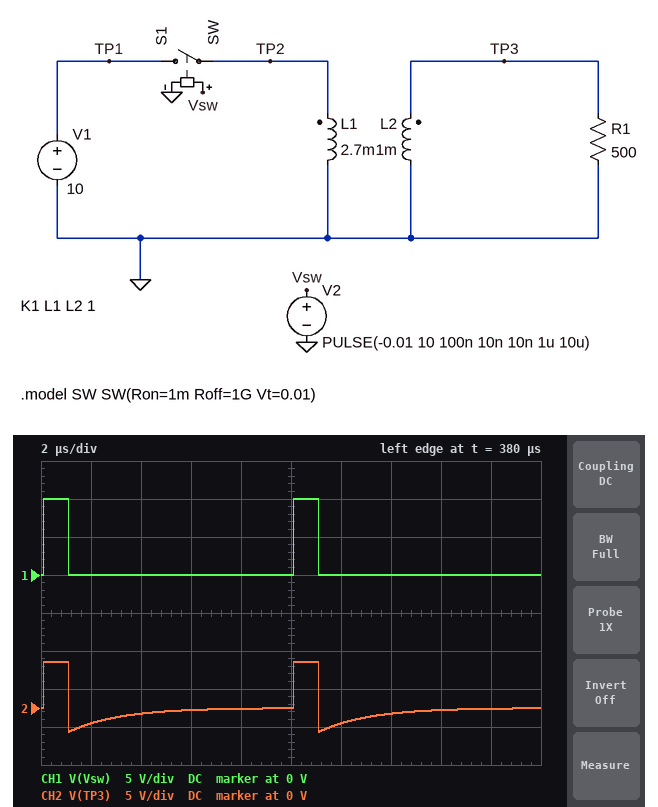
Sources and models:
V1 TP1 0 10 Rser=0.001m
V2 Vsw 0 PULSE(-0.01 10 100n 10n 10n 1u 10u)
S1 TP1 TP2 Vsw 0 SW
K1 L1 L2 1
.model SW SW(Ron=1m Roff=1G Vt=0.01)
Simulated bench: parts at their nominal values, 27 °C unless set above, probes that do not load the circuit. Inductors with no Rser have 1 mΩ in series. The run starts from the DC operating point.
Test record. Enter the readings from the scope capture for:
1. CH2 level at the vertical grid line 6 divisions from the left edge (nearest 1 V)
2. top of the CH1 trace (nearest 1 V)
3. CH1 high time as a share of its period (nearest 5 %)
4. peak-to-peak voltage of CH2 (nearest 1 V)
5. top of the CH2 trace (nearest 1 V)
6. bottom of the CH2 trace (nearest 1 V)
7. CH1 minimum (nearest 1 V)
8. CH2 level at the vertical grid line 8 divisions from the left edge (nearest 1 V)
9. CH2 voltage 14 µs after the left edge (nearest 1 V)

-2 V
10 V
10 %
9 V
6 V
-3 V
0 V
0 V
-1 V
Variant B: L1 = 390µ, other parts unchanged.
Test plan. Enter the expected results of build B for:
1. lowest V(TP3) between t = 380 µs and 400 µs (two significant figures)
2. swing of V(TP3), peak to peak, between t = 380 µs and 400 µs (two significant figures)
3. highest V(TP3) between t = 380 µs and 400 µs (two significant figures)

-8.3 V
24 V
16 V
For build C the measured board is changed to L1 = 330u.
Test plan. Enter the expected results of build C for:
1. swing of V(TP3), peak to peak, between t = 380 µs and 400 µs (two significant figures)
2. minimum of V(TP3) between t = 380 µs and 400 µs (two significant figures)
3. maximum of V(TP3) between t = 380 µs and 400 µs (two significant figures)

26 V
-9.0 V
17 V
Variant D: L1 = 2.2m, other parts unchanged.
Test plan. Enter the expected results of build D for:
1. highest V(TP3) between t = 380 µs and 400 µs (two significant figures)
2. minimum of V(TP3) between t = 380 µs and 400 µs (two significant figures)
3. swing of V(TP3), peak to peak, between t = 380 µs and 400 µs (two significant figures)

6.7 V
-3.5 V
10 V
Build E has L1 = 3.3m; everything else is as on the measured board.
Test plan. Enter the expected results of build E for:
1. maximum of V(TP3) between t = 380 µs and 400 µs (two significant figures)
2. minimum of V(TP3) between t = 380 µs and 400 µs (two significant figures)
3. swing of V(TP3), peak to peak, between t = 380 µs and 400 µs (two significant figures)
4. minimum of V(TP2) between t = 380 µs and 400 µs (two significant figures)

5.5 V
-2.8 V
8.3 V
-5.2 V
